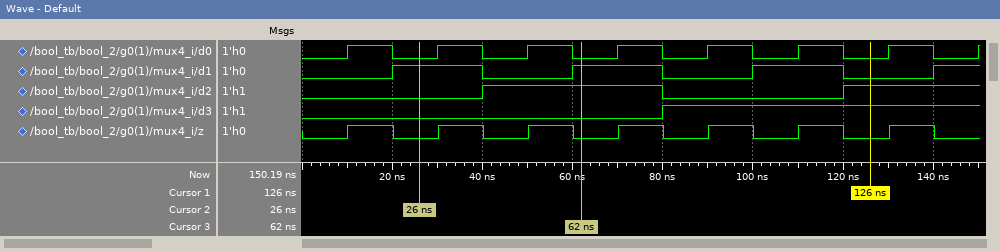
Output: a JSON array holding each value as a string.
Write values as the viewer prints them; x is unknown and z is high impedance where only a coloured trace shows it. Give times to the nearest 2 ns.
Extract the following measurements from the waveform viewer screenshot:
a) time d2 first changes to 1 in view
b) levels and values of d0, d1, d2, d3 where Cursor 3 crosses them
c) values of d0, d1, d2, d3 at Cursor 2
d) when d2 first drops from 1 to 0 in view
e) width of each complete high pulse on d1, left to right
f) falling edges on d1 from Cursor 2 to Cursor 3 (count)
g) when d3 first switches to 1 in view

["40 ns", "d0=0, d1=1, d2=1, d3=0", "d0=0, d1=1, d2=0, d3=0", "80 ns", "20 ns, 20 ns, 20 ns", "1", "80 ns"]
